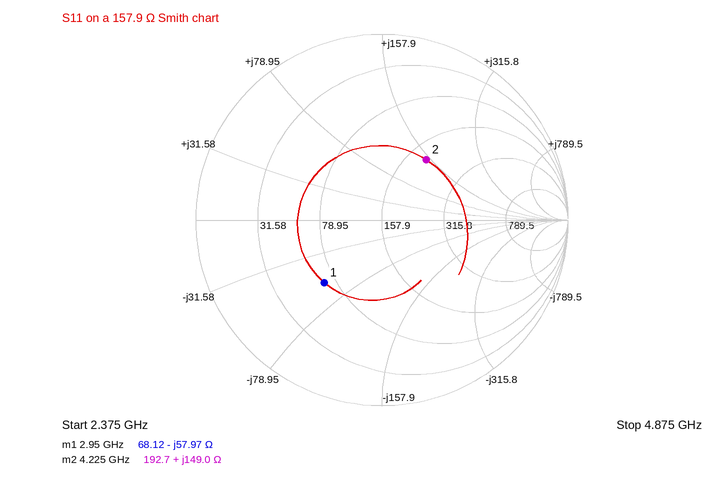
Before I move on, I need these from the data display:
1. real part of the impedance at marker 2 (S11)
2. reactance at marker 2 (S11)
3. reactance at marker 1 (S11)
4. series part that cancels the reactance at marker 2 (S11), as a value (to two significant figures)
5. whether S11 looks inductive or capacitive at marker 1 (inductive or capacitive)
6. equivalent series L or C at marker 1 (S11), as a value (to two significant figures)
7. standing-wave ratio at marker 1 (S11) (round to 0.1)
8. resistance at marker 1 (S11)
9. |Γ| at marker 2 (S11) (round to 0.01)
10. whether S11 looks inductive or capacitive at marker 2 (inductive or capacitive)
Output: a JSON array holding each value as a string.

["192.7 Ω", "+149.0 Ω", "-57.97 Ω", "250 fF", "capacitive", "930 fF", "2.7", "68.12 Ω", "0.40", "inductive"]
